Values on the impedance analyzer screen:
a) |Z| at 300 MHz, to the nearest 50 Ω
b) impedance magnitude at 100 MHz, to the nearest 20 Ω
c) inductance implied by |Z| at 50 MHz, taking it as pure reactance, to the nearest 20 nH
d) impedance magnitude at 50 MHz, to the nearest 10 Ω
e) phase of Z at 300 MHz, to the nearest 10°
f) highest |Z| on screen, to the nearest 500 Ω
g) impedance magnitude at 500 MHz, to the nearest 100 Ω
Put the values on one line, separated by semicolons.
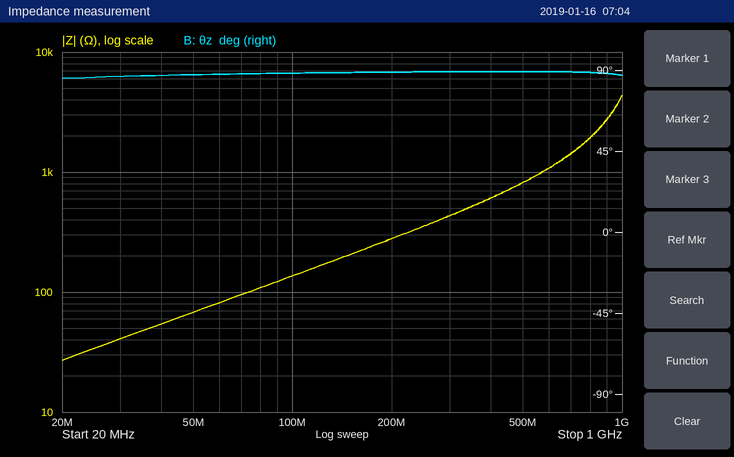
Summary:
450 Ω; 140 Ω; 220 nH; 70 Ω; 90°; 4.5 kΩ; 800 Ω
